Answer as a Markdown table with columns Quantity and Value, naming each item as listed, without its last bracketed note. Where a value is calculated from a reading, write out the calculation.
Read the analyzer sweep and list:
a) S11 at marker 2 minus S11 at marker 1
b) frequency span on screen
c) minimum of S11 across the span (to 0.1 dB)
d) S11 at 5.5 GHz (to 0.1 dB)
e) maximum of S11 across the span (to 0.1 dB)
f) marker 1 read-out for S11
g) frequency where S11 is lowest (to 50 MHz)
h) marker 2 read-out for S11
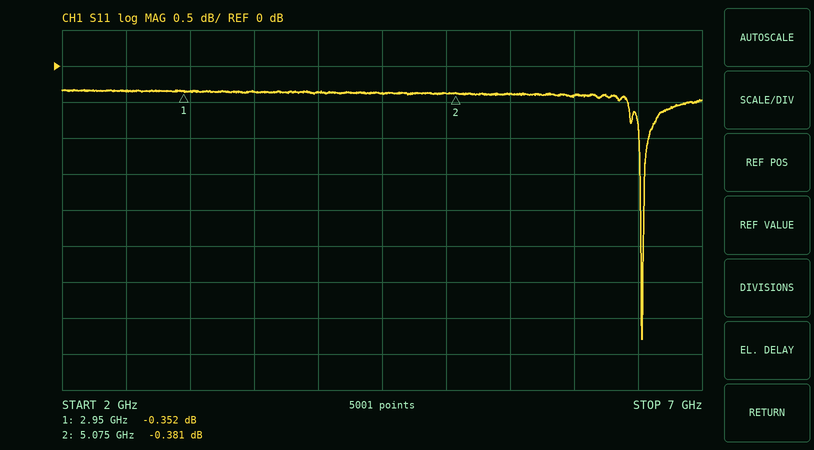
| Quantity | Value |
|---|---|
| S11 at marker 2 minus S11 at marker 1 | -0.381 − (-0.352) = -0.029 dB |
| frequency span on screen | 5 GHz |
| minimum of S11 across the span | -3.8 dB |
| S11 at 5.5 GHz | -0.4 dB |
| maximum of S11 across the span | -0.3 dB |
| marker 1 read-out for S11 | -0.352 dB |
| frequency where S11 is lowest | 6.55 GHz |
| marker 2 read-out for S11 | -0.381 dB |
